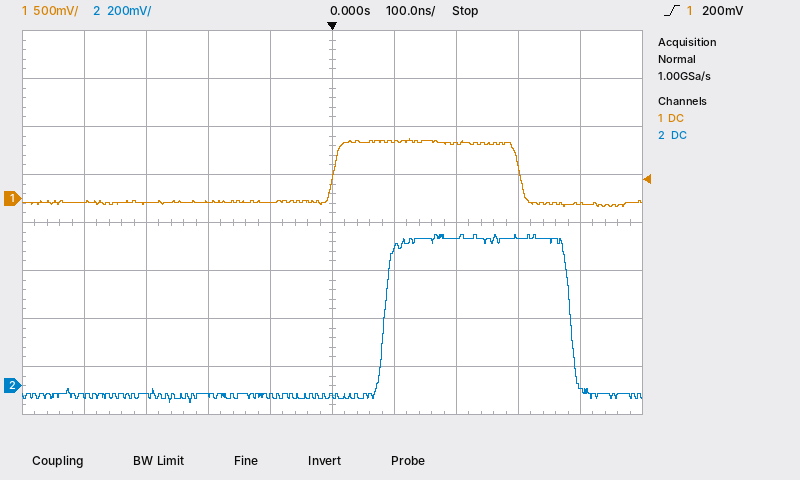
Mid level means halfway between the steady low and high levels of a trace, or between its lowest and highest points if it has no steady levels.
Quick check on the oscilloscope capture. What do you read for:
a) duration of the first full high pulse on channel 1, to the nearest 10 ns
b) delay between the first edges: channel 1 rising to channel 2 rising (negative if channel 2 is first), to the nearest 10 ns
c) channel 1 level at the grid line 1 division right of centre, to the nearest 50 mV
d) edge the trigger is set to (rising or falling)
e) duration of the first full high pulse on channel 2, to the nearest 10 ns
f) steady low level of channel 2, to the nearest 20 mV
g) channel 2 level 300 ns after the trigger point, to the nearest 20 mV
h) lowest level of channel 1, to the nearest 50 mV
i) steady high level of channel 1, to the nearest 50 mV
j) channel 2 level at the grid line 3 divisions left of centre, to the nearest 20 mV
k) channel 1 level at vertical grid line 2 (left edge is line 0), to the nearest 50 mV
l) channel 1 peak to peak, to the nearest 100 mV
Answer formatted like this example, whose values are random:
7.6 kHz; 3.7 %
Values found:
300 ns; +80 ns; 600 mV; rising; 300 ns; -40 mV; 620 mV; -100 mV; 600 mV; -40 mV; -50 mV; 700 mV
